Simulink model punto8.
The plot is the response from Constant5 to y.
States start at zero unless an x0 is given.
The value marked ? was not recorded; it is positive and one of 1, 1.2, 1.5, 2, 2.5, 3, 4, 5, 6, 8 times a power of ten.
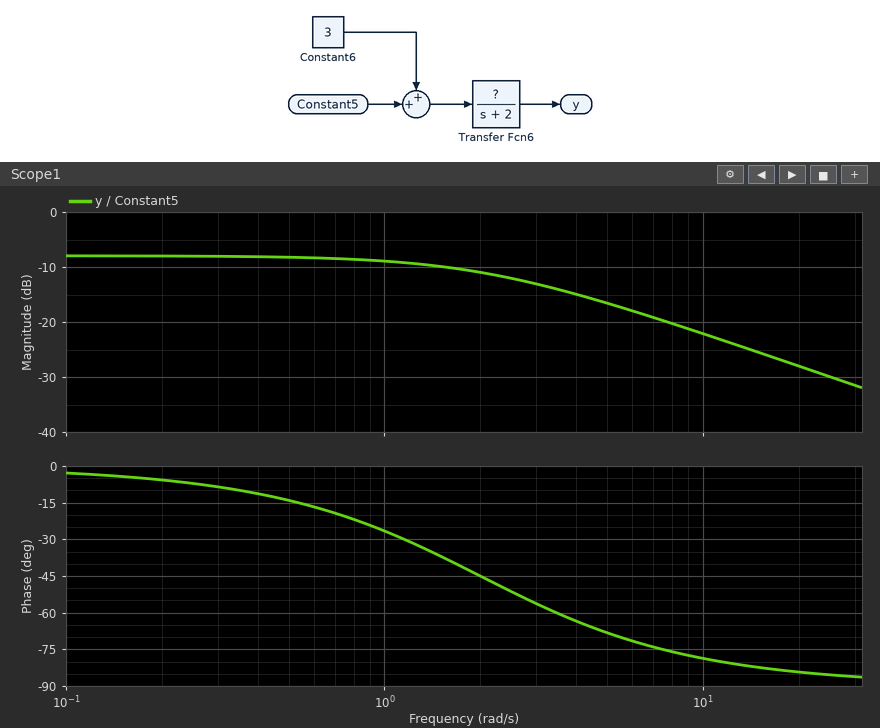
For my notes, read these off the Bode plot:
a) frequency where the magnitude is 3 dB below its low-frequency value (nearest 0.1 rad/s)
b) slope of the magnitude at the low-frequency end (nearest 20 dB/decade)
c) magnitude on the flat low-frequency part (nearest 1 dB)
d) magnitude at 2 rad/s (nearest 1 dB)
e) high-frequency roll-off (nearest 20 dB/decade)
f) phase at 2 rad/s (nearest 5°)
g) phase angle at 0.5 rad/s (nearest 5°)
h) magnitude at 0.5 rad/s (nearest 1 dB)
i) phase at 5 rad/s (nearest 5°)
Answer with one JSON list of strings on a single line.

["2.0 rad/s", "0 dB/decade", "-8 dB", "-11 dB", "-20 dB/decade", "-45°", "-15°", "-8 dB", "-70°"]
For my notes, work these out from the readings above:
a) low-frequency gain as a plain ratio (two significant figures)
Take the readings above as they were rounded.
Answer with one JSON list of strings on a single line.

["0.40"]
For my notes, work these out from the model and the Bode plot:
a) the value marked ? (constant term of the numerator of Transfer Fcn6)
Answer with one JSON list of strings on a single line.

["0.8"]
